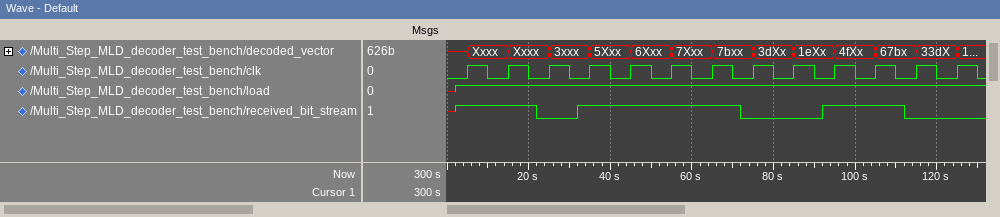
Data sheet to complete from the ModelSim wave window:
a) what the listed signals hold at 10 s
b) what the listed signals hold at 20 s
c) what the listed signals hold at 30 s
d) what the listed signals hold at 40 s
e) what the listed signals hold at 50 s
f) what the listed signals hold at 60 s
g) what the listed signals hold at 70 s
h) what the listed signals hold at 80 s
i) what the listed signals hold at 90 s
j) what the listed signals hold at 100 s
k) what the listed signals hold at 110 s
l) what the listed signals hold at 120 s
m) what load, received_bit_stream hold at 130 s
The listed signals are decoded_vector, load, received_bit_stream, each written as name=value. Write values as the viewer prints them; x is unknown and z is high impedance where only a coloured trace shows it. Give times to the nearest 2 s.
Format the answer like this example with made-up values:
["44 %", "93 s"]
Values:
["decoded_vector=Xxxx, load=1, received_bit_stream=1", "decoded_vector=Xxxx, load=1, received_bit_stream=1", "decoded_vector=3xxx, load=1, received_bit_stream=0", "decoded_vector=5Xxx, load=1, received_bit_stream=1", "decoded_vector=6Xxx, load=1, received_bit_stream=1", "decoded_vector=7Xxx, load=1, received_bit_stream=1", "decoded_vector=7bxx, load=1, received_bit_stream=1", "decoded_vector=3dXx, load=1, received_bit_stream=0", "decoded_vector=1eXx, load=1, received_bit_stream=0", "decoded_vector=4fXx, load=1, received_bit_stream=1", "decoded_vector=67bx, load=1, received_bit_stream=1", "decoded_vector=33dX, load=1, received_bit_stream=0", "load=1, received_bit_stream=0"]
